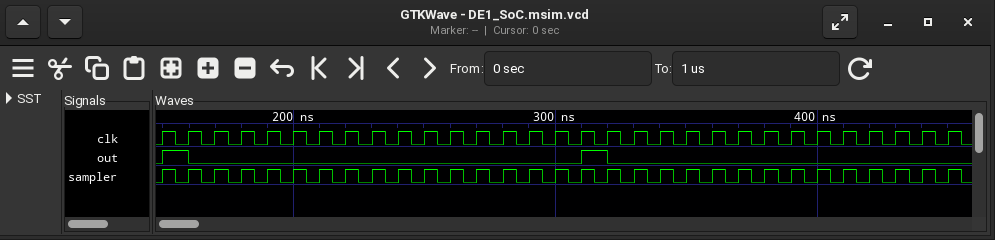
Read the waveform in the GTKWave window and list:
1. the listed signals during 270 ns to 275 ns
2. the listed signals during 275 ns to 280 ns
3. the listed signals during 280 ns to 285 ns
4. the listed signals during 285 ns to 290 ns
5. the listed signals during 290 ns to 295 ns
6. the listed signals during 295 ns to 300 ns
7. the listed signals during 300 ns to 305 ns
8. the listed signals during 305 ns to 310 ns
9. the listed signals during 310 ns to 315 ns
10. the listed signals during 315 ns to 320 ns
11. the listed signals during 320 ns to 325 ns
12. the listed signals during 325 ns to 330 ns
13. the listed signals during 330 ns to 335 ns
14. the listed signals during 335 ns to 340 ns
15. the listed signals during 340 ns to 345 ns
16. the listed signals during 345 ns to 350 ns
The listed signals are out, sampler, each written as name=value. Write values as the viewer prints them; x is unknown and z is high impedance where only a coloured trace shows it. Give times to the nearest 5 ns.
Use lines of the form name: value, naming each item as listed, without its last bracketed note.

the listed signals during 270 ns to 275 ns: out=0, sampler=1
the listed signals during 275 ns to 280 ns: out=0, sampler=0
the listed signals during 280 ns to 285 ns: out=0, sampler=1
the listed signals during 285 ns to 290 ns: out=0, sampler=0
the listed signals during 290 ns to 295 ns: out=0, sampler=1
the listed signals during 295 ns to 300 ns: out=0, sampler=0
the listed signals during 300 ns to 305 ns: out=0, sampler=1
the listed signals during 305 ns to 310 ns: out=0, sampler=0
the listed signals during 310 ns to 315 ns: out=1, sampler=1
the listed signals during 315 ns to 320 ns: out=1, sampler=0
the listed signals during 320 ns to 325 ns: out=0, sampler=1
the listed signals during 325 ns to 330 ns: out=0, sampler=0
the listed signals during 330 ns to 335 ns: out=0, sampler=1
the listed signals during 335 ns to 340 ns: out=0, sampler=0
the listed signals during 340 ns to 345 ns: out=0, sampler=1
the listed signals during 345 ns to 350 ns: out=0, sampler=0
